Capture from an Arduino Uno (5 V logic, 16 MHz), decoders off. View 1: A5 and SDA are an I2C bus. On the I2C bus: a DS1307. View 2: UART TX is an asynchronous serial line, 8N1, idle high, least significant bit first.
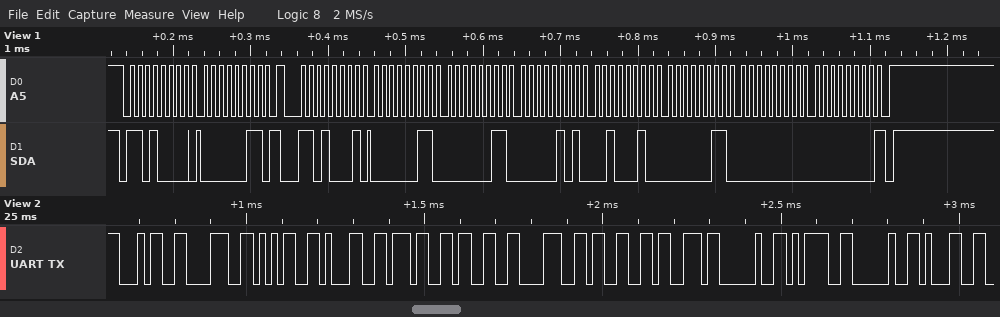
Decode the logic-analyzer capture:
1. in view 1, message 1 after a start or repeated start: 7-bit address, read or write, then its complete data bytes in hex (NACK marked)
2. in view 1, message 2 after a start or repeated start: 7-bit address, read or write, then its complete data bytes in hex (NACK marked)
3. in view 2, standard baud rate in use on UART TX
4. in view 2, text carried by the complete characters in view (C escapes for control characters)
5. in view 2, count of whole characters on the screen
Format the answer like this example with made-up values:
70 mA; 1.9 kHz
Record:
0x68 write: 03; 0x68 read: 03 03 05 22 03 00 00 NACK; 57600 baud; "48517383s = 1"; 13
